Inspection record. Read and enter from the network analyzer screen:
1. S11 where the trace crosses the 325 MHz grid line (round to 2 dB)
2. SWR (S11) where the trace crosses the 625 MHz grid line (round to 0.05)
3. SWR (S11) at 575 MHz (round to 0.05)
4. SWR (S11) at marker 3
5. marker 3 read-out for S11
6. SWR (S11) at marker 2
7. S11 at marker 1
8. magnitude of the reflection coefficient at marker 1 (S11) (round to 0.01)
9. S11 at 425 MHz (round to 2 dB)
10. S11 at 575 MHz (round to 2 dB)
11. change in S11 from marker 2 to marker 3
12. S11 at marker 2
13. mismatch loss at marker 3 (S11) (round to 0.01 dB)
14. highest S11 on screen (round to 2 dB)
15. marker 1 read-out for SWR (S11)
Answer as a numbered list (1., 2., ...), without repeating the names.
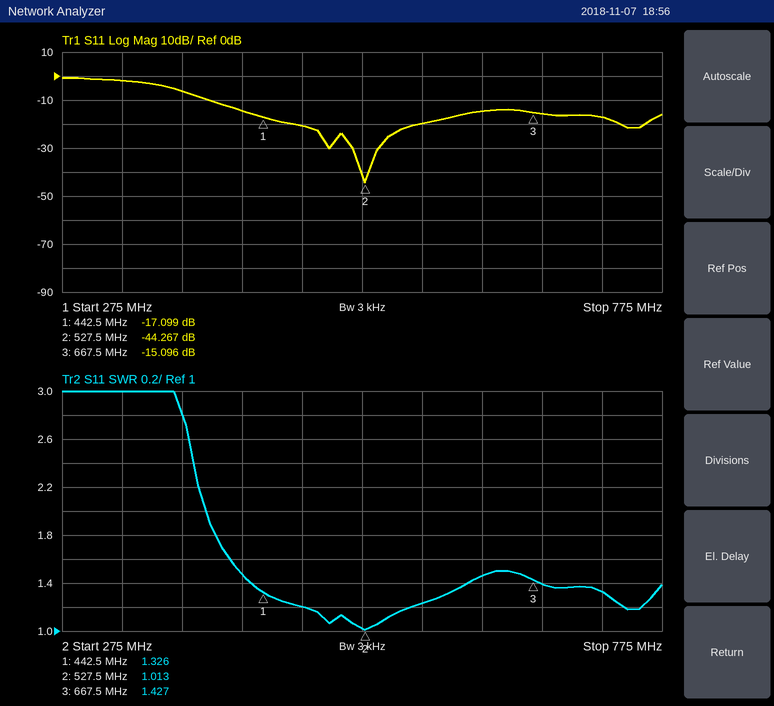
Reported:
1. -2 dB
2. 1.45
3. 1.25
4. 1.427
5. -15.096 dB
6. 1.013
7. -17.099 dB
8. 0.14
9. -14 dB
10. -20 dB
11. 29.171 dB
12. -44.267 dB
13. 0.14 dB
14. 0 dB
15. 1.326
